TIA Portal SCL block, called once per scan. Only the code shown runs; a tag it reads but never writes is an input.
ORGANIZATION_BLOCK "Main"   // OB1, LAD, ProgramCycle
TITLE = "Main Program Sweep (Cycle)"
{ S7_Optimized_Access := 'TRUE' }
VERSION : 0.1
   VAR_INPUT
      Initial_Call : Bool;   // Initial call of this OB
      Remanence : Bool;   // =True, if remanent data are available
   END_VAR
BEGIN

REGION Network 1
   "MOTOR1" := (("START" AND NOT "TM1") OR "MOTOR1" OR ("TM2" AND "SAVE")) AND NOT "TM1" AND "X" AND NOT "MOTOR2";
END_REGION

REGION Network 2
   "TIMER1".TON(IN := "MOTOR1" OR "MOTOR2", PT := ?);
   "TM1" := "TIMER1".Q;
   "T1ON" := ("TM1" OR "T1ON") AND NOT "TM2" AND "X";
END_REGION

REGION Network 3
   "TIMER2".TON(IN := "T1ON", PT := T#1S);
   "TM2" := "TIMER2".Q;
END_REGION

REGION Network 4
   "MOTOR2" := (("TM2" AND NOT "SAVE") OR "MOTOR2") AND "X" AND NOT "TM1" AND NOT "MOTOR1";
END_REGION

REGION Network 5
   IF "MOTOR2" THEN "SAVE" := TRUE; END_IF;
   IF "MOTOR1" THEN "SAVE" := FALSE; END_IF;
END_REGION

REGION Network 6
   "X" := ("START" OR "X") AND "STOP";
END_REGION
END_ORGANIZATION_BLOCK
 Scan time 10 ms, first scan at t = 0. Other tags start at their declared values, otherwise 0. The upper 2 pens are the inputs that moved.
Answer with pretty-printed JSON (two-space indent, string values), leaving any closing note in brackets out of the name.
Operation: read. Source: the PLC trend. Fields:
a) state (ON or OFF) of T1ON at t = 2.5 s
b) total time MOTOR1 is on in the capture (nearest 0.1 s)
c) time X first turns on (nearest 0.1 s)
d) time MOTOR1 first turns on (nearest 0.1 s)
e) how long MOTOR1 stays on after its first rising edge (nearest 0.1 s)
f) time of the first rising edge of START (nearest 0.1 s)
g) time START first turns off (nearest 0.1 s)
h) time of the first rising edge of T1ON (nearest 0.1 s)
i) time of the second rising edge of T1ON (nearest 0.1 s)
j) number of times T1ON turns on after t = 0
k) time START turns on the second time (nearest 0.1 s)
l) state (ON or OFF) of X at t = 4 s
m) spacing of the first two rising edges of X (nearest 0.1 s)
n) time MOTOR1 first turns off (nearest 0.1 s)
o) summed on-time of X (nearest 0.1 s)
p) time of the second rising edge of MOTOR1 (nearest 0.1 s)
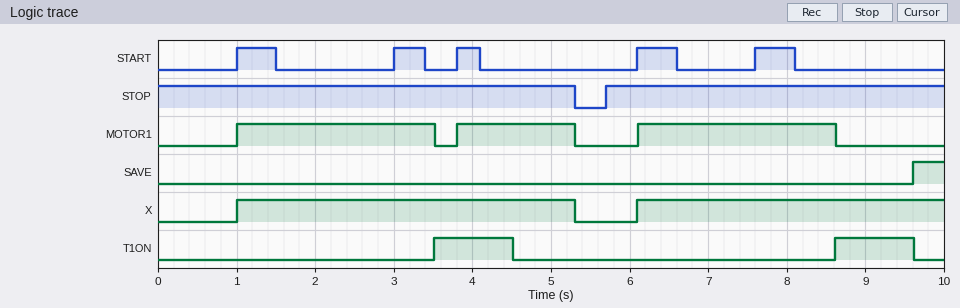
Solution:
{
  "state (ON or OFF) of T1ON at t = 2.5 s": "OFF",
  "total time MOTOR1 is on in the capture": "6.5 s",
  "time X first turns on": "1.0 s",
  "time MOTOR1 first turns on": "1.0 s",
  "how long MOTOR1 stays on after its first rising edge": "2.5 s",
  "time of the first rising edge of START": "1.0 s",
  "time START first turns off": "1.5 s",
  "time of the first rising edge of T1ON": "3.5 s",
  "time of the second rising edge of T1ON": "8.6 s",
  "number of times T1ON turns on after t = 0": "2",
  "time START turns on the second time": "3.0 s",
  "state (ON or OFF) of X at t = 4 s": "ON",
  "spacing of the first two rising edges of X": "5.1 s",
  "time MOTOR1 first turns off": "3.5 s",
  "summed on-time of X": "8.2 s",
  "time of the second rising edge of MOTOR1": "3.8 s"
}
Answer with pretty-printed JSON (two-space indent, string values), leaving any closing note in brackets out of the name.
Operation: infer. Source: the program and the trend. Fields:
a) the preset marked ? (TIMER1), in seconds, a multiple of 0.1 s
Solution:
{
  "the preset marked ? (TIMER1), in seconds, a multiple of 0.1 s": "2.5 s"
}
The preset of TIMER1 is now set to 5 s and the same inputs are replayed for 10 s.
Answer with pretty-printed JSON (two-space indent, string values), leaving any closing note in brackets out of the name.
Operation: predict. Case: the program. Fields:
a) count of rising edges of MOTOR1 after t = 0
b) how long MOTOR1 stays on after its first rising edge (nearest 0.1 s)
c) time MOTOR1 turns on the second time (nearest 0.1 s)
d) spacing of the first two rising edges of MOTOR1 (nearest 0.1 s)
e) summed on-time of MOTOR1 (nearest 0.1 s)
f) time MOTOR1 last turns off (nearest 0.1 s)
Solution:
{
  "count of rising edges of MOTOR1 after t = 0": "2",
  "how long MOTOR1 stays on after its first rising edge": "4.3 s",
  "time MOTOR1 turns on the second time": "6.1 s",
  "spacing of the first two rising edges of MOTOR1": "5.1 s",
  "summed on-time of MOTOR1": "8.2 s",
  "time MOTOR1 last turns off": "5.3 s"
}
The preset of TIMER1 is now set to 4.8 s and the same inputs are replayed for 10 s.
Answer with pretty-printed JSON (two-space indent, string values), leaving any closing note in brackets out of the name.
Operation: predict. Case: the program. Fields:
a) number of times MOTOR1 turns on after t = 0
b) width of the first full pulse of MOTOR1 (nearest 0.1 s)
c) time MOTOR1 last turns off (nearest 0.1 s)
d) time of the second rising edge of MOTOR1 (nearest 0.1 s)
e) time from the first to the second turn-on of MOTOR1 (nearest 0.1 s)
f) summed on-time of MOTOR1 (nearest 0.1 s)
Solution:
{
  "number of times MOTOR1 turns on after t = 0": "2",
  "width of the first full pulse of MOTOR1": "4.3 s",
  "time MOTOR1 last turns off": "5.3 s",
  "time of the second rising edge of MOTOR1": "6.1 s",
  "time from the first to the second turn-on of MOTOR1": "5.1 s",
  "summed on-time of MOTOR1": "8.2 s"
}
